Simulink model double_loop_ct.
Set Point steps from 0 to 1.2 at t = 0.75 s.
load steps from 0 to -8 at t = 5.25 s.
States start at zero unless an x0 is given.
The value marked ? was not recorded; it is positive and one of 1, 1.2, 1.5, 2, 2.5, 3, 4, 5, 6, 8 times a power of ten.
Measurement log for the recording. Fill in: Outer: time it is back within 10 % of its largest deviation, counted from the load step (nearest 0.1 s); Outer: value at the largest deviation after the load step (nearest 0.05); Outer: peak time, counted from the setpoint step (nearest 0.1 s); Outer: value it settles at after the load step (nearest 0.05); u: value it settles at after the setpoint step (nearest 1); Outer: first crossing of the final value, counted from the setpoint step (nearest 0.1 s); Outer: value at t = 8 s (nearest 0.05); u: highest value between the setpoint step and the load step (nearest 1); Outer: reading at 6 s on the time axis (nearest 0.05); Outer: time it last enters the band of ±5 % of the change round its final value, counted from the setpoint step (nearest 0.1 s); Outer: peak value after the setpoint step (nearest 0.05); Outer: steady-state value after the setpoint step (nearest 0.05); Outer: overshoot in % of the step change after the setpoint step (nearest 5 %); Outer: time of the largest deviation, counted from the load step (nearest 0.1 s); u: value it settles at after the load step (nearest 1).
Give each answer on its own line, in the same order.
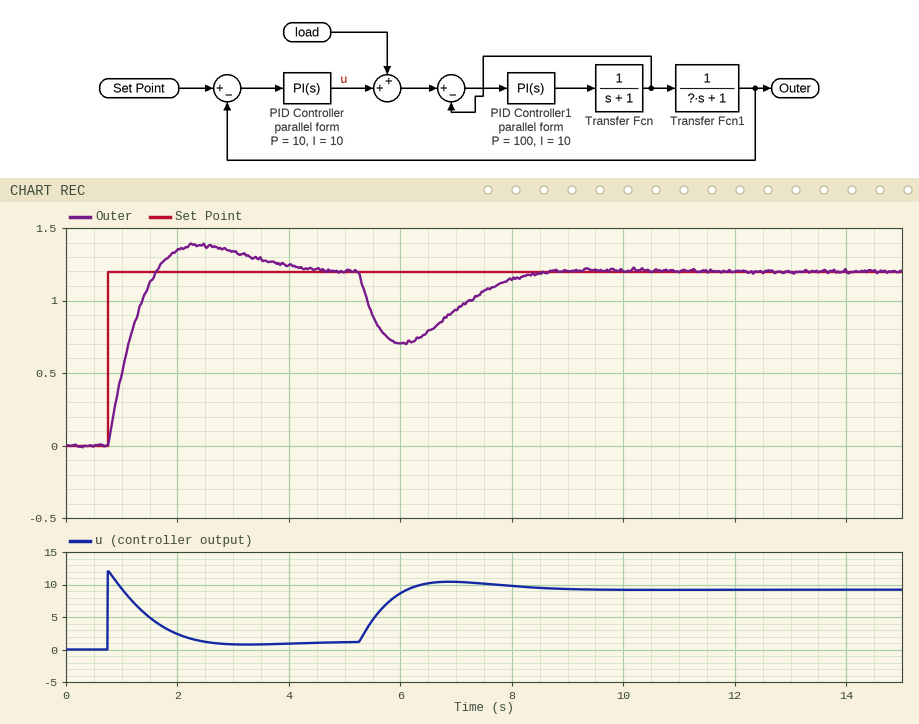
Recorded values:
2.8 s
0.70
1.6 s
1.20
1
0.9 s
1.15
12
0.70
3.0 s
1.40
1.20
15 %
0.8 s
9
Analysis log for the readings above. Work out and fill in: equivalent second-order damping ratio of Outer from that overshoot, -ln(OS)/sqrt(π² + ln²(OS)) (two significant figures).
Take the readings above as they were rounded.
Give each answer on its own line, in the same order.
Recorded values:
0.52
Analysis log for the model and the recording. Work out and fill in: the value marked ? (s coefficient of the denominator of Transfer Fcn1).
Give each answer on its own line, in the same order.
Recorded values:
5
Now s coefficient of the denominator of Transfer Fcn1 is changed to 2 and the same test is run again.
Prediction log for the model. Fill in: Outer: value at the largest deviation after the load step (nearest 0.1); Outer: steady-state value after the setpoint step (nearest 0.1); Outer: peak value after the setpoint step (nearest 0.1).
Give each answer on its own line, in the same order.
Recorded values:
0.6
1.2
1.3
